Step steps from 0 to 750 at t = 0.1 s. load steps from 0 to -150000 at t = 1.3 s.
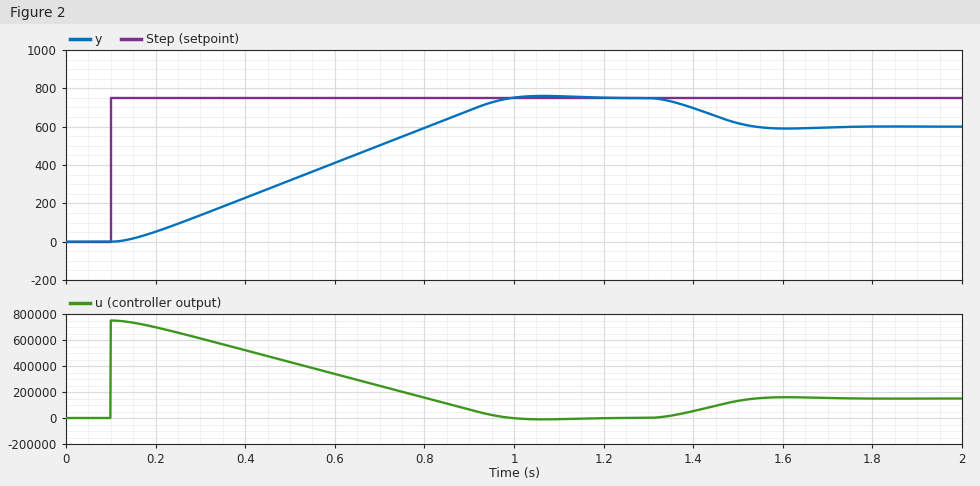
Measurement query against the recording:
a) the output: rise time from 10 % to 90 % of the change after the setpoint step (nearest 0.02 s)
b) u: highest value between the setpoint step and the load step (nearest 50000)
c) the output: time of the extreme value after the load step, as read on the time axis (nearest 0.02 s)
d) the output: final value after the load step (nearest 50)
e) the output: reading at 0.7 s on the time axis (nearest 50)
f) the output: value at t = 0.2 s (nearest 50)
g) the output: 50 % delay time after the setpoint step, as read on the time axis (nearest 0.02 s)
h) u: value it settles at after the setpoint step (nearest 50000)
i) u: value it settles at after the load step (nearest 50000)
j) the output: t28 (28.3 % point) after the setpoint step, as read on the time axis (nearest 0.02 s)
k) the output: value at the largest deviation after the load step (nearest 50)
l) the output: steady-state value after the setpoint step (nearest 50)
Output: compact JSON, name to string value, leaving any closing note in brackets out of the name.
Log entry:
{"the output: rise time from 10 % to 90 % of the change after the setpoint step": "0.66 s", "u: highest value between the setpoint step and the load step": "750000", "the output: time of the extreme value after the load step, as read on the time axis": "1.60 s", "the output: final value after the load step": "600", "the output: reading at 0.7 s on the time axis": "500", "the output: value at t = 0.2 s": "50", "the output: 50 % delay time after the setpoint step, as read on the time axis": "0.56 s", "u: value it settles at after the setpoint step": "0", "u: value it settles at after the load step": "150000", "the output: t28 (28.3 % point) after the setpoint step, as read on the time axis": "0.38 s", "the output: value at the largest deviation after the load step": "600", "the output: steady-state value after the setpoint step": "750"}
